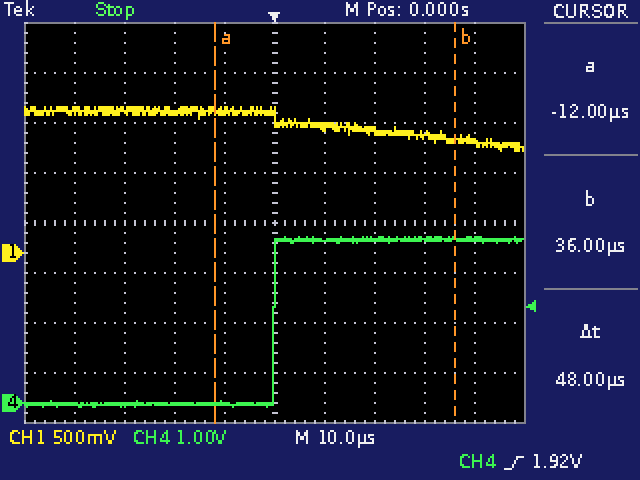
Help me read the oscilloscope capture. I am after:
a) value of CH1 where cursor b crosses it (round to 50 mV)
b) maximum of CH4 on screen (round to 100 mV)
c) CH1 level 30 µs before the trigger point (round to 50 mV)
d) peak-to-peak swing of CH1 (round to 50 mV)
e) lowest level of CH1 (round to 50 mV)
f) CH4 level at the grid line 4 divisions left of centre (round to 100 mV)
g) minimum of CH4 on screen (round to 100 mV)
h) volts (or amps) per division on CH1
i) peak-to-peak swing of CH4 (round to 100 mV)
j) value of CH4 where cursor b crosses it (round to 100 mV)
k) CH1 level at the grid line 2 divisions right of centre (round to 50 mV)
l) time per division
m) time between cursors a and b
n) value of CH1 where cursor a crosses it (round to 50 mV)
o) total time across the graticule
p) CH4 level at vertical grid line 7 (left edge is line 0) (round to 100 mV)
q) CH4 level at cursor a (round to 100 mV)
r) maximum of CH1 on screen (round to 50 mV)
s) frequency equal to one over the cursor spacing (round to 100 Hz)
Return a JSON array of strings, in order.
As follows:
["1.15 V", "3.3 V", "1.40 V", "450 mV", "1.00 V", "0.0 V", "-100 mV", "500 mV", "3.4 V", "3.3 V", "1.20 V", "10 µs", "48 µs", "1.40 V", "100 µs", "3.3 V", "0.0 V", "1.45 V", "20.8 kHz"]
